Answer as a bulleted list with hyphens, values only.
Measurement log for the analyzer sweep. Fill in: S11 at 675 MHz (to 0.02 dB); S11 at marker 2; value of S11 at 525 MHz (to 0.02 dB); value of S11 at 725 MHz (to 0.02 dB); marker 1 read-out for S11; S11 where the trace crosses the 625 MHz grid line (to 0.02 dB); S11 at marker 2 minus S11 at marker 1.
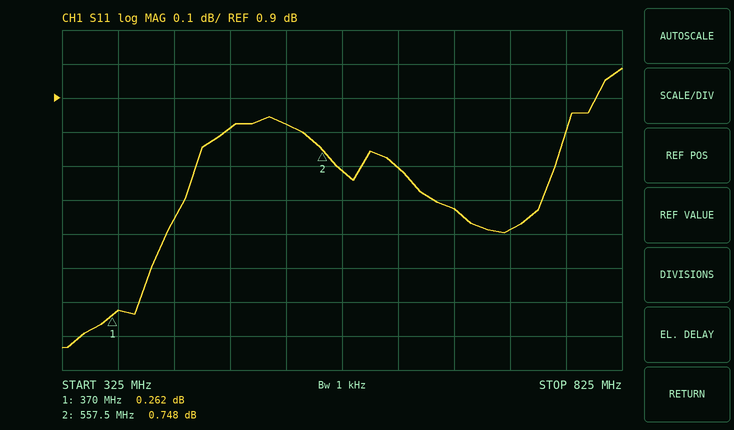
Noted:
- 0.58 dB
- 0.748 dB
- 0.82 dB
- 0.52 dB
- 0.262 dB
- 0.70 dB
- 0.486 dB
